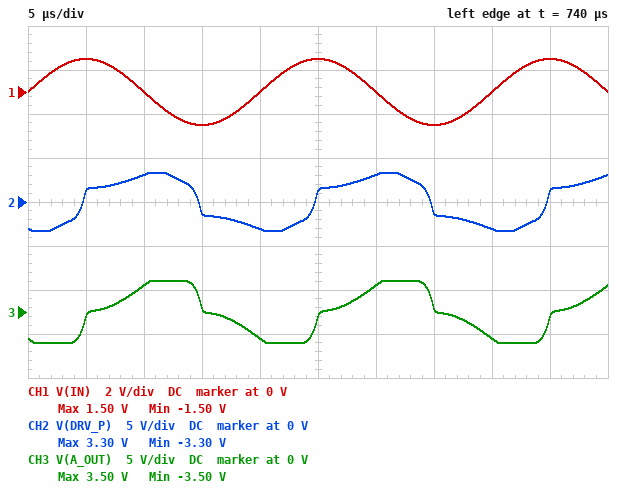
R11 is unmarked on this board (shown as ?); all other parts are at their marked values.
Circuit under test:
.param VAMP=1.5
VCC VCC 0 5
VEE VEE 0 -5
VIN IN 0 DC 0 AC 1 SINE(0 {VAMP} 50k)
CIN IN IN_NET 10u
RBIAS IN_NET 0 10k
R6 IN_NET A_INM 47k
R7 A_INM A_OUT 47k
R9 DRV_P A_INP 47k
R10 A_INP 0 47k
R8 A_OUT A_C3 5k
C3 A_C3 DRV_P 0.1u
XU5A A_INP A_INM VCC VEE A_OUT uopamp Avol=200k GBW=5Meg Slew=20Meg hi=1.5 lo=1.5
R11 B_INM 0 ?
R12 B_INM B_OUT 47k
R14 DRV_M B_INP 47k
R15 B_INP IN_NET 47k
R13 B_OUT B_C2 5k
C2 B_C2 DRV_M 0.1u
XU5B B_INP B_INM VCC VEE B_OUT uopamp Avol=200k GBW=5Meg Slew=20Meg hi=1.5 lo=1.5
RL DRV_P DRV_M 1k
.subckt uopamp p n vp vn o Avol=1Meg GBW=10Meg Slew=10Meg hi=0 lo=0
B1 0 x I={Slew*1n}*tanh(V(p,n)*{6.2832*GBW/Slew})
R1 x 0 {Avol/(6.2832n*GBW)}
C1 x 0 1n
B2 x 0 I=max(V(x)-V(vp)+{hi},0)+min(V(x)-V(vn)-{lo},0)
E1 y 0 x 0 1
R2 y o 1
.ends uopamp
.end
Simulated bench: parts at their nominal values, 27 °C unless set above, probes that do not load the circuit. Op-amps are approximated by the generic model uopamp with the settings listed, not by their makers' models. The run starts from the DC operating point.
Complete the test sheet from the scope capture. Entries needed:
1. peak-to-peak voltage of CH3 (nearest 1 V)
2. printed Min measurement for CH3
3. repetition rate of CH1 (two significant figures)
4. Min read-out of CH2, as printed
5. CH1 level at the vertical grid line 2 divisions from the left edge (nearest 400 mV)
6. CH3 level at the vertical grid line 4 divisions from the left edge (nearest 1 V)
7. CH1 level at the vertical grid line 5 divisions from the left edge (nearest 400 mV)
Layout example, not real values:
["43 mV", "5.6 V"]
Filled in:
["7 V", "-3.50 V", "50 kHz", "-3.30 V", "0 V", "-3 V", "1.6 V"]
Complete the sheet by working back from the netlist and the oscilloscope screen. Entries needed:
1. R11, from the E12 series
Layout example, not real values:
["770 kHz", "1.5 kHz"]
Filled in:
["27 kΩ"]
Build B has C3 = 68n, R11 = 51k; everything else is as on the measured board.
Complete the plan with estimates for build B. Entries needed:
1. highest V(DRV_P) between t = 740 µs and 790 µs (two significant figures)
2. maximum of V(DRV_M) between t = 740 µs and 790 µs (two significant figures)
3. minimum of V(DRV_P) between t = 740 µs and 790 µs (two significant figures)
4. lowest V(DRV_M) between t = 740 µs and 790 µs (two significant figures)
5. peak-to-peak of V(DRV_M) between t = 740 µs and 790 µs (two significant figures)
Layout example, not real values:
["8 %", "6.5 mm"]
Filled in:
["66 mV", "240 mV", "-71 mV", "-250 mV", "490 mV"]
